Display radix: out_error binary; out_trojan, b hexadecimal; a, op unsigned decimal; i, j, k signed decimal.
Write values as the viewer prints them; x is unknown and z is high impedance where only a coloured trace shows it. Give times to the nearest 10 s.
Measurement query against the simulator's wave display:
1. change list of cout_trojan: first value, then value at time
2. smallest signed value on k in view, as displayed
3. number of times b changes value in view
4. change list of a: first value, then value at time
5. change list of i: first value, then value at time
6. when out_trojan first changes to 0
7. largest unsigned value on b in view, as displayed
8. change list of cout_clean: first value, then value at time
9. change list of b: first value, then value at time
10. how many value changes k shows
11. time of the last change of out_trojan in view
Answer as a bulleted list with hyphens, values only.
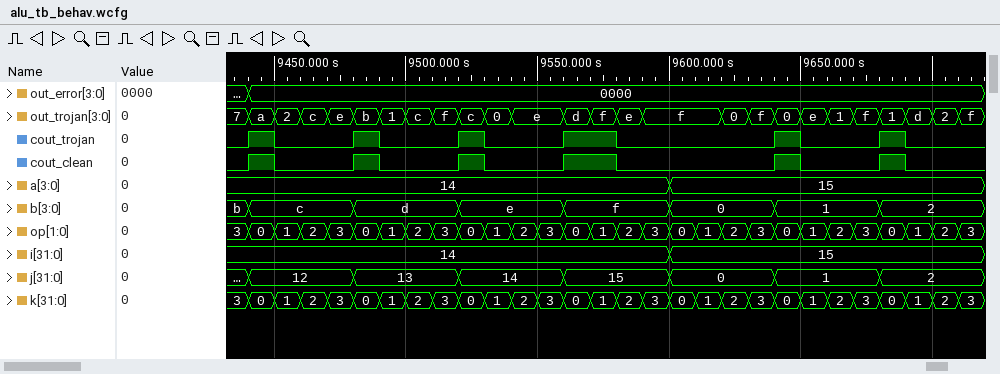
- 0, 1 at 9440 s, 0 at 9450 s, 1 at 9480 s, 0 at 9490 s, 1 at 9520 s, 0 at 9530 s, 1 at 9560 s, 0 at 9580 s, 1 at 9640 s, 0 at 9650 s, 1 at 9680 s, 0 at 9690 s
- 0
- 7
- 14, 15 at 9600 s
- 14, 15 at 9600 s
- 9530 s
- f
- 0, 1 at 9440 s, 0 at 9450 s, 1 at 9480 s, 0 at 9490 s, 1 at 9520 s, 0 at 9530 s, 1 at 9560 s, 0 at 9580 s, 1 at 9640 s, 0 at 9650 s, 1 at 9680 s, 0 at 9690 s
- b, c at 9440 s, d at 9480 s, e at 9520 s, f at 9560 s, 0 at 9600 s, 1 at 9640 s, 2 at 9680 s
- 28
- 9710 s
